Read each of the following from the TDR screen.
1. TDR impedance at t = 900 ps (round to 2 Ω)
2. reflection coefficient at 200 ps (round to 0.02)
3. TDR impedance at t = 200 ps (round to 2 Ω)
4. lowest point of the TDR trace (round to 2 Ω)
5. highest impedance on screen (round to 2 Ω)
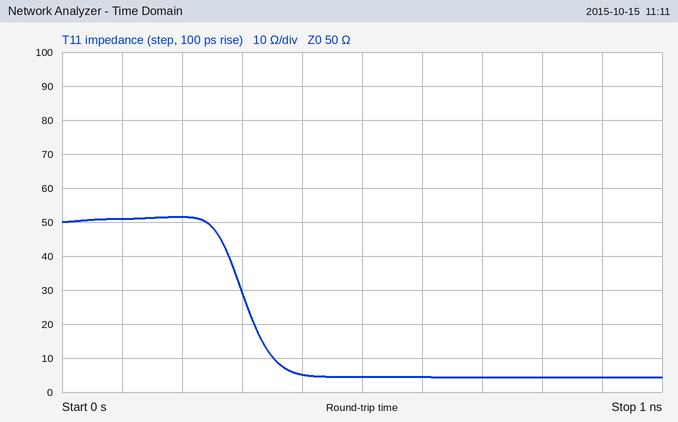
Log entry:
4 Ω
+0.02
52 Ω
4 Ω
52 Ω
